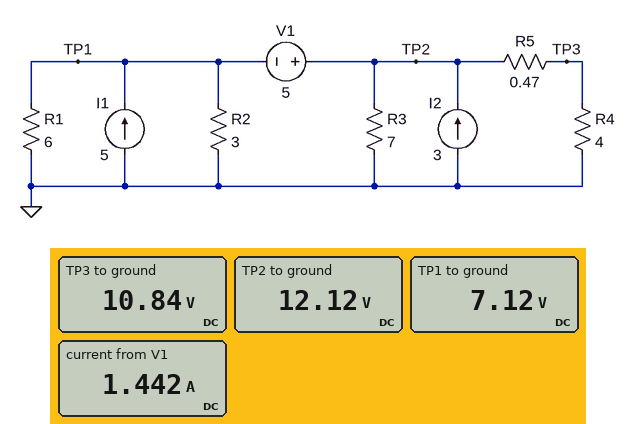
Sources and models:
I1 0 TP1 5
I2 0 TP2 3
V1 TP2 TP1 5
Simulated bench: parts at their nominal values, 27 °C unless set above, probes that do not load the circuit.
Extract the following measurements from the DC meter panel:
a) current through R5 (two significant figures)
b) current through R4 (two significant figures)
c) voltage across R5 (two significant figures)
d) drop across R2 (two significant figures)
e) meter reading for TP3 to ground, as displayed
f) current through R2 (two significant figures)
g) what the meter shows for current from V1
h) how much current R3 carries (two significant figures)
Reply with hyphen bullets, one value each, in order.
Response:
- 2.7 A
- 2.7 A
- 1.3 V
- 7.1 V
- 10.84 V
- 2.4 A
- 1.442 A
- 1.7 A
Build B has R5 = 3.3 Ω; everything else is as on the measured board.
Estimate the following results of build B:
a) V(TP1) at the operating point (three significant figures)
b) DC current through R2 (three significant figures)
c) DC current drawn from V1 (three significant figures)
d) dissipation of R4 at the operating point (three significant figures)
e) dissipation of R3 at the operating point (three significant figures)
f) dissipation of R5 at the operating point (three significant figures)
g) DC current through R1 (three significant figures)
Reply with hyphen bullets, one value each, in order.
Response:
- 8.46 V
- 2.82 A
- 768 mA
- 13.6 W
- 25.9 W
- 11.2 W
- 1.41 A
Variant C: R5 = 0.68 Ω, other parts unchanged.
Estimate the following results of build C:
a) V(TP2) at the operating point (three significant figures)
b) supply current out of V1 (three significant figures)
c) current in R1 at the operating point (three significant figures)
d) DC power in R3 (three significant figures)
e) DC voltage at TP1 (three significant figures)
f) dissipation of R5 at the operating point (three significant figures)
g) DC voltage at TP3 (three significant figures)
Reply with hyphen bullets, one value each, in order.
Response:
- 12.3 V
- 1.37 A
- 1.21 A
- 21.5 W
- 7.26 V
- 4.67 W
- 10.5 V
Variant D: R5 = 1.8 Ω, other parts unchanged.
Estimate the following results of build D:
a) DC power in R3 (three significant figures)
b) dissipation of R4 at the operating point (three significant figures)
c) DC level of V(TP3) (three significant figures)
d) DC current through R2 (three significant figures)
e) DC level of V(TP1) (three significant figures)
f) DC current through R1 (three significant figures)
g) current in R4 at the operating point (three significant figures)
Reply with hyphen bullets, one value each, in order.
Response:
- 23.7 W
- 19.7 W
- 8.88 V
- 2.63 A
- 7.88 V
- 1.31 A
- 2.22 A
